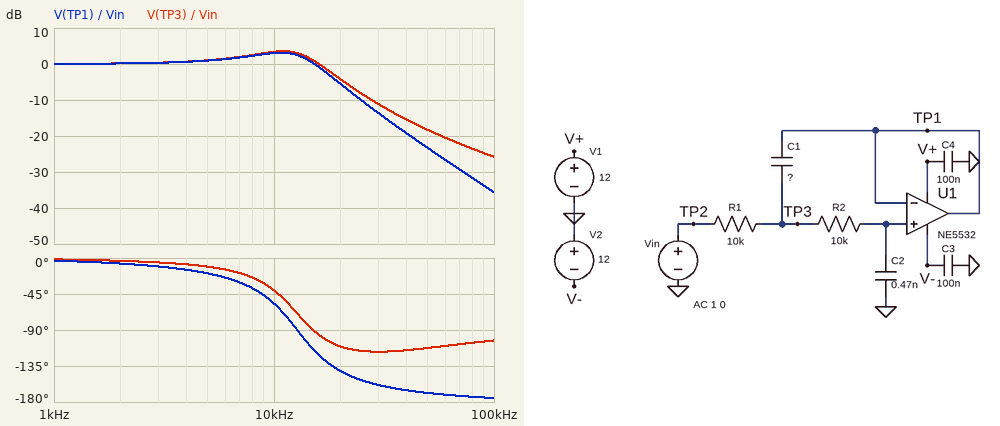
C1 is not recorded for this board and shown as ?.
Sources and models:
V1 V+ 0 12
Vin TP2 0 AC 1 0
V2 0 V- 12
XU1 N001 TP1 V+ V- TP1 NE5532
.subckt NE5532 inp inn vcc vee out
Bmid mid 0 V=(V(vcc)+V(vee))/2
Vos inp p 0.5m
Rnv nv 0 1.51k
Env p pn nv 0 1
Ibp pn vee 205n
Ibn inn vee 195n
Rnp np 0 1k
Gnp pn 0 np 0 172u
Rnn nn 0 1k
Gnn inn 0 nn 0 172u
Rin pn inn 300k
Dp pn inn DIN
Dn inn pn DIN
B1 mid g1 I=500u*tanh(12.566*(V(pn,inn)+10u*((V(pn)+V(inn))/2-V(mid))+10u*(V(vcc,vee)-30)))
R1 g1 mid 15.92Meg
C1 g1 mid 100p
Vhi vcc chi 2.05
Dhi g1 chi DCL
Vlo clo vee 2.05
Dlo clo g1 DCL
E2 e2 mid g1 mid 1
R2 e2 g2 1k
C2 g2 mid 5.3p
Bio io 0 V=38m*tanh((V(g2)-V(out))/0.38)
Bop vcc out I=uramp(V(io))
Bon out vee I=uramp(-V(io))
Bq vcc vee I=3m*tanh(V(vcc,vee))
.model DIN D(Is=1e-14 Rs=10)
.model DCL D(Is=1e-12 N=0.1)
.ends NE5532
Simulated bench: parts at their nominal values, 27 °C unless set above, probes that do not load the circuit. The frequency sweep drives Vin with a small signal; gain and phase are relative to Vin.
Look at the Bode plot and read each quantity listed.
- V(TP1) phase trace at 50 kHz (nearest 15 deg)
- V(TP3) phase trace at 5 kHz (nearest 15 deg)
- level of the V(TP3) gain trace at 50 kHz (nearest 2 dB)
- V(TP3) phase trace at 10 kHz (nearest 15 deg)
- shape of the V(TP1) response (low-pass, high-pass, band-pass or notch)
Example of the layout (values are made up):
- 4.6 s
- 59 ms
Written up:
- -165 deg
- -15 deg
- -18 dB
- -45 deg
- low-pass
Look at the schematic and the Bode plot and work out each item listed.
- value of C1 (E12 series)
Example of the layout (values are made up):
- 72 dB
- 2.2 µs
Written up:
- 3.3 nF
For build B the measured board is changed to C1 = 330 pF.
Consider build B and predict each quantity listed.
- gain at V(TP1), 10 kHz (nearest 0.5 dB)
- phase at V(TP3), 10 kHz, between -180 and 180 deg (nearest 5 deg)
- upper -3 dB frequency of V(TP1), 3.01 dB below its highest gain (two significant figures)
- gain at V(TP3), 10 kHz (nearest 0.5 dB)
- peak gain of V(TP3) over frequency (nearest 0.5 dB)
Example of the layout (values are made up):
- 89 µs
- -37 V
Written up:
- -1.0 dB
- -15 deg
- 20 kHz
- -0.5 dB
- 0 dB
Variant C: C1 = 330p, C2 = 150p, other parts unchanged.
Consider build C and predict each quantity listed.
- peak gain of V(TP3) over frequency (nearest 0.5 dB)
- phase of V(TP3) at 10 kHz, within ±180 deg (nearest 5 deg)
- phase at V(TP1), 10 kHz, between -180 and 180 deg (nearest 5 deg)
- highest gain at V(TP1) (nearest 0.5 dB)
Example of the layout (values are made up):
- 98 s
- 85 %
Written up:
- 0.5 dB
- -5 deg
- -10 deg
- 0 dB
